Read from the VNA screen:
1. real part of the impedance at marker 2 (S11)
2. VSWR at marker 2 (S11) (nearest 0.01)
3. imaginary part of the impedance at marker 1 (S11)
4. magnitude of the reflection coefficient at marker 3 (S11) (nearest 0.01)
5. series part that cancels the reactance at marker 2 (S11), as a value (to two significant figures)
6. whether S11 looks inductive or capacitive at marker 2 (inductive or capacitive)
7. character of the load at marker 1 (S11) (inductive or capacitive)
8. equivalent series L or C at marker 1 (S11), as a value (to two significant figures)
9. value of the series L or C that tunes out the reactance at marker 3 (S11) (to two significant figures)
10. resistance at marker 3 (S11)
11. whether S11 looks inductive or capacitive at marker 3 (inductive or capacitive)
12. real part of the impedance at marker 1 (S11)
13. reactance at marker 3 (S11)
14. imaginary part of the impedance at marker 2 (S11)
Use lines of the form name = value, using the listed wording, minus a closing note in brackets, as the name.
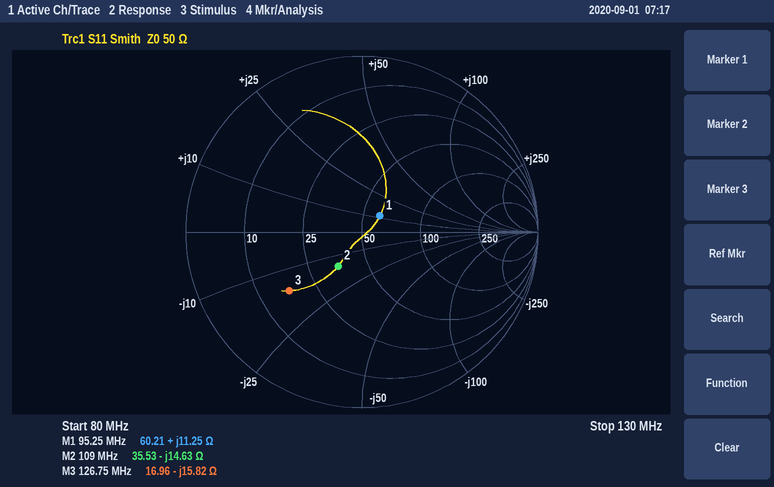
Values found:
real part of the impedance at marker 2 = 35.53 Ω
VSWR at marker 2 (S11) = 1.62
imaginary part of the impedance at marker 1 = +11.25 Ω
magnitude of the reflection coefficient at marker 3 (S11) = 0.53
series part that cancels the reactance at marker 2 (S11), as a value = 21 nH
whether S11 looks inductive or capacitive at marker 2 = capacitive
character of the load at marker 1 (S11) = inductive
equivalent series L or C at marker 1 (S11), as a value = 19 nH
value of the series L or C that tunes out the reactance at marker 3 (S11) = 20 nH
resistance at marker 3 = 16.96 Ω
whether S11 looks inductive or capacitive at marker 3 = capacitive
real part of the impedance at marker 1 = 60.21 Ω
reactance at marker 3 = -15.82 Ω
imaginary part of the impedance at marker 2 = -14.63 Ω
